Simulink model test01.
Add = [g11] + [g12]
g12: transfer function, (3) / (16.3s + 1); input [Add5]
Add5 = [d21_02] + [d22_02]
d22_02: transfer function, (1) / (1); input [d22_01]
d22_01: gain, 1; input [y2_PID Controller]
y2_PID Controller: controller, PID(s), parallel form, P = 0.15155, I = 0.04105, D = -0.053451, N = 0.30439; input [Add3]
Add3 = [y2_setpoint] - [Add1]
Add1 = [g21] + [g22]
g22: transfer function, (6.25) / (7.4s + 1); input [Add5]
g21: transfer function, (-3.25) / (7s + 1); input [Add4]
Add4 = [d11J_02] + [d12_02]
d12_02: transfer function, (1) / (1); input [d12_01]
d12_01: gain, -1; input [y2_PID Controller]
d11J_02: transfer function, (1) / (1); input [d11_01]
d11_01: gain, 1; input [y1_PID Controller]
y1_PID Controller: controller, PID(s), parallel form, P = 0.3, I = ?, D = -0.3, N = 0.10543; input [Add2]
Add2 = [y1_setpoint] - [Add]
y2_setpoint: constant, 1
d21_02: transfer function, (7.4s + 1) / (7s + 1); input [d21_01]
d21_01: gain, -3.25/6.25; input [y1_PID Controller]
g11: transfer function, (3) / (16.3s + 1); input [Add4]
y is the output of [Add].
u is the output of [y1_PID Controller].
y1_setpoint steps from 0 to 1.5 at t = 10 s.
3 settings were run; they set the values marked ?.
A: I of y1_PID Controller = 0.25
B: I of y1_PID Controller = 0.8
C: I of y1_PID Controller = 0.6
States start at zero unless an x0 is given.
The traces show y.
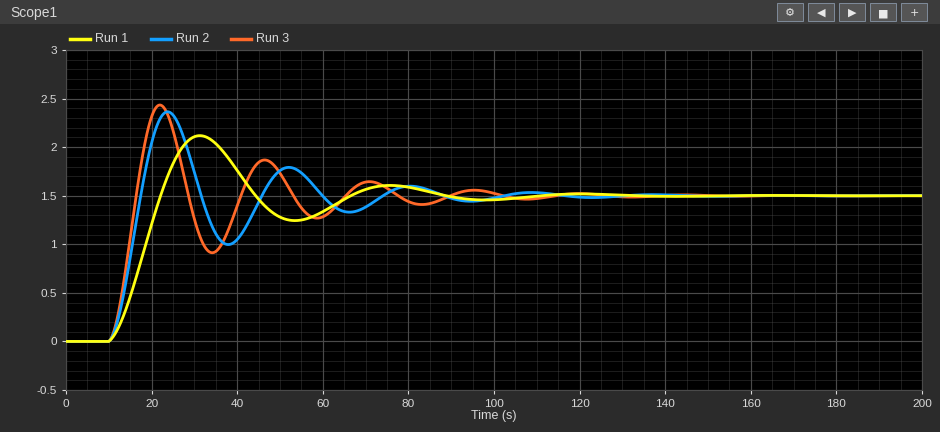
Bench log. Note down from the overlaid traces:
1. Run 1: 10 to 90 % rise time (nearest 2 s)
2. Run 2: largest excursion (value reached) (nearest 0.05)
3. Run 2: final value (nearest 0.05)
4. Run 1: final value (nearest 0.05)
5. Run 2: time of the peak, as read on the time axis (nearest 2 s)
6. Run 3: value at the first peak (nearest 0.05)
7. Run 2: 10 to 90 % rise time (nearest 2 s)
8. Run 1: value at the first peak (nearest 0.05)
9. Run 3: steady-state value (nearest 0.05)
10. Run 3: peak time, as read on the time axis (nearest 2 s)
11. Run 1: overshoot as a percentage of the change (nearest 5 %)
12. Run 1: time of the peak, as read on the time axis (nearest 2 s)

8 s
2.35
1.50
1.50
24 s
2.45
6 s
2.10
1.50
22 s
40 %
32 s
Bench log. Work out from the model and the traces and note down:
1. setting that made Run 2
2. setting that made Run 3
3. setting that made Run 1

C
B
A
